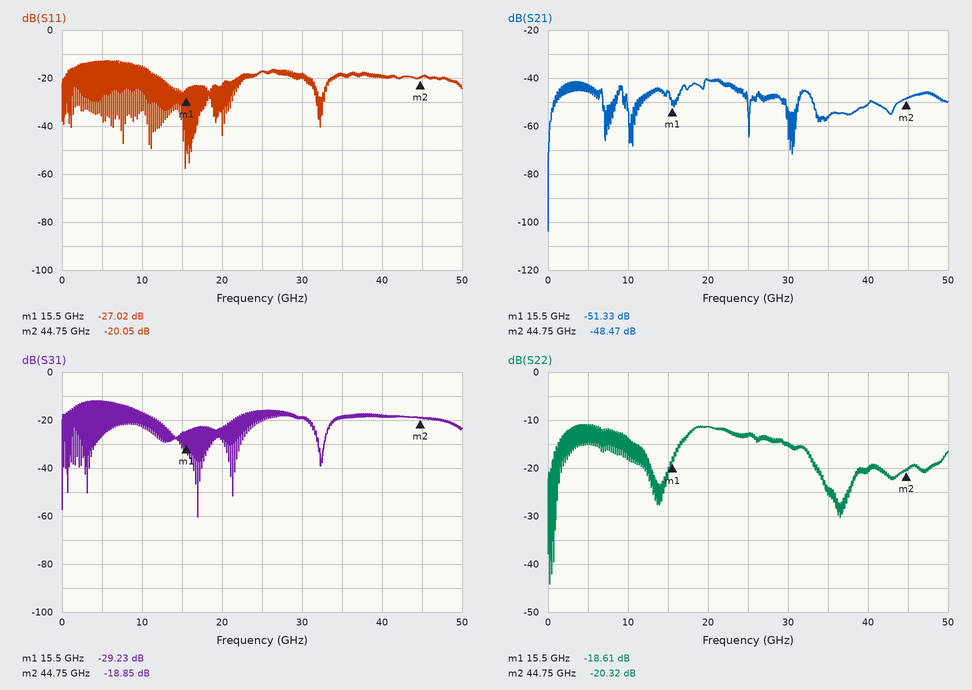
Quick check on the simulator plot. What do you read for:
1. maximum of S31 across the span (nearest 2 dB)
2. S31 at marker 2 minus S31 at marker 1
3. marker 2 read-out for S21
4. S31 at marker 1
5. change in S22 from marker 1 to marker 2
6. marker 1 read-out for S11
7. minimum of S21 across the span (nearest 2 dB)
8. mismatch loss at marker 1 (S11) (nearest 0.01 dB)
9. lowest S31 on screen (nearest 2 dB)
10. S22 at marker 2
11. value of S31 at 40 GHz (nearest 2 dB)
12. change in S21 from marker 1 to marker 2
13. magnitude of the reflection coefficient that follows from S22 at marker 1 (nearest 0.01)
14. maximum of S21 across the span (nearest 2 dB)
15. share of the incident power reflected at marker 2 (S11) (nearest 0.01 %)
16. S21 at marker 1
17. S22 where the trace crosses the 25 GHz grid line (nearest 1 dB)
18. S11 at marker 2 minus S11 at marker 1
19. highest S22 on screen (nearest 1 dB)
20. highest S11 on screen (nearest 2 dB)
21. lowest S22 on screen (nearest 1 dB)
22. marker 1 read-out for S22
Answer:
-12 dB
10.38 dB
-48.47 dB
-29.23 dB
-1.71 dB
-27.02 dB
-104 dB
0.01 dB
-60 dB
-20.32 dB
-18 dB
2.86 dB
0.12
-40 dB
0.99 %
-51.33 dB
-13 dB
6.97 dB
-11 dB
-12 dB
-44 dB
-18.61 dB
